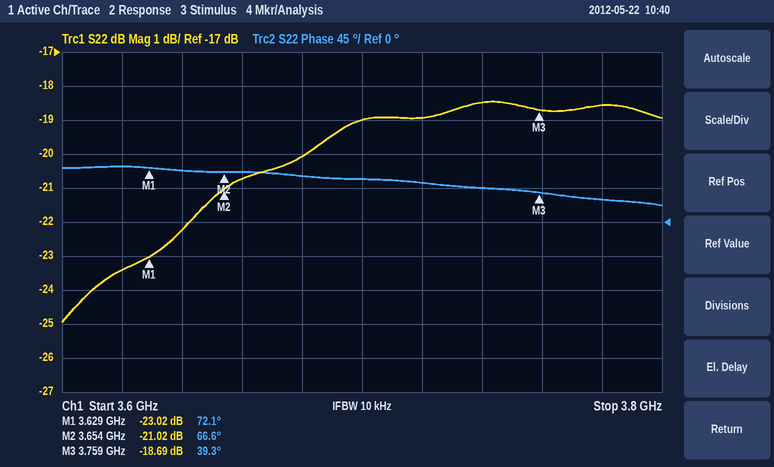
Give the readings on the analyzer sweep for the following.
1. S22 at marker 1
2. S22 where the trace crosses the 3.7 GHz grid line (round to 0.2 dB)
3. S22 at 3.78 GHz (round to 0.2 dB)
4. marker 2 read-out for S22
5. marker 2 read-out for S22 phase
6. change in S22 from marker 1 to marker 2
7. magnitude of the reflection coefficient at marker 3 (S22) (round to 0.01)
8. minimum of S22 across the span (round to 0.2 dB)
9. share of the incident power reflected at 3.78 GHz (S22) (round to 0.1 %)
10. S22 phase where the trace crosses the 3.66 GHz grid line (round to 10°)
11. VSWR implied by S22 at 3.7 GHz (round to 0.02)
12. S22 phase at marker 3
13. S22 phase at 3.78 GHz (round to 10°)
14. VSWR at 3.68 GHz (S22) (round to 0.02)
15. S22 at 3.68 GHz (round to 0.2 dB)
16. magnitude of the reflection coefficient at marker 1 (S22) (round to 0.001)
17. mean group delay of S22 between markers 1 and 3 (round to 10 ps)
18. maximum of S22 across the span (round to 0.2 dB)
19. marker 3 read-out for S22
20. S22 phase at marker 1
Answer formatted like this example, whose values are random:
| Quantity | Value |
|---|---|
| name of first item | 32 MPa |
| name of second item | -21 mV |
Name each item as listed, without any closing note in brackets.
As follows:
| Quantity | Value |
|---|---|
| S22 at marker 1 | -23.02 dB |
| S22 where the trace crosses the 3.7 GHz grid line | -19.0 dB |
| S22 at 3.78 GHz | -18.6 dB |
| marker 2 read-out for S22 | -21.02 dB |
| marker 2 read-out for S22 phase | 66.6° |
| change in S22 from marker 1 to marker 2 | 2.00 dB |
| magnitude of the reflection coefficient at marker 3 (S22) | 0.12 |
| minimum of S22 across the span | -25.0 dB |
| share of the incident power reflected at 3.78 GHz (S22) | 1.4 % |
| S22 phase where the trace crosses the 3.66 GHz grid line | 70° |
| VSWR implied by S22 at 3.7 GHz | 1.26 |
| S22 phase at marker 3 | 39.3° |
| S22 phase at 3.78 GHz | 30° |
| VSWR at 3.68 GHz (S22) | 1.22 |
| S22 at 3.68 GHz | -20.0 dB |
| magnitude of the reflection coefficient at marker 1 (S22) | 0.071 |
| mean group delay of S22 between markers 1 and 3 | 700 ps |
| maximum of S22 across the span | -18.4 dB |
| marker 3 read-out for S22 | -18.69 dB |
| S22 phase at marker 1 | 72.1° |
